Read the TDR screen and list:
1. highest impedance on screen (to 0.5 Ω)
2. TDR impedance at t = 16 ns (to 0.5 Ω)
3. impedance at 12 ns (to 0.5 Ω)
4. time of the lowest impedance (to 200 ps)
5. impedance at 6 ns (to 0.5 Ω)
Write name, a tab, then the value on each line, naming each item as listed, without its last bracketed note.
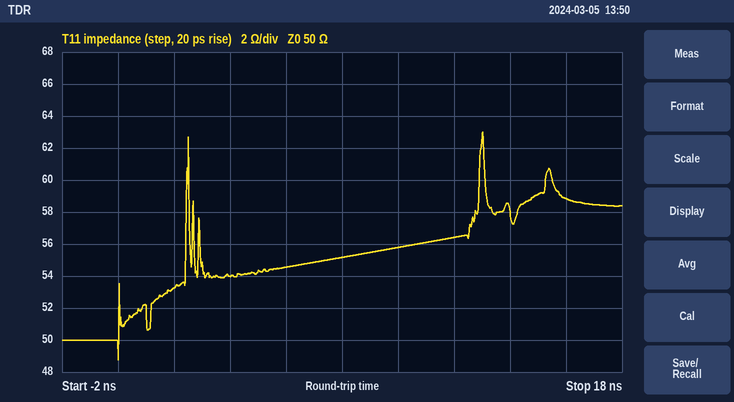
highest impedance on screen	63.0 Ω
TDR impedance at t = 16 ns	59.0 Ω
impedance at 12 ns	56.5 Ω
time of the lowest impedance	0.0 ns
impedance at 6 ns	54.5 Ω
